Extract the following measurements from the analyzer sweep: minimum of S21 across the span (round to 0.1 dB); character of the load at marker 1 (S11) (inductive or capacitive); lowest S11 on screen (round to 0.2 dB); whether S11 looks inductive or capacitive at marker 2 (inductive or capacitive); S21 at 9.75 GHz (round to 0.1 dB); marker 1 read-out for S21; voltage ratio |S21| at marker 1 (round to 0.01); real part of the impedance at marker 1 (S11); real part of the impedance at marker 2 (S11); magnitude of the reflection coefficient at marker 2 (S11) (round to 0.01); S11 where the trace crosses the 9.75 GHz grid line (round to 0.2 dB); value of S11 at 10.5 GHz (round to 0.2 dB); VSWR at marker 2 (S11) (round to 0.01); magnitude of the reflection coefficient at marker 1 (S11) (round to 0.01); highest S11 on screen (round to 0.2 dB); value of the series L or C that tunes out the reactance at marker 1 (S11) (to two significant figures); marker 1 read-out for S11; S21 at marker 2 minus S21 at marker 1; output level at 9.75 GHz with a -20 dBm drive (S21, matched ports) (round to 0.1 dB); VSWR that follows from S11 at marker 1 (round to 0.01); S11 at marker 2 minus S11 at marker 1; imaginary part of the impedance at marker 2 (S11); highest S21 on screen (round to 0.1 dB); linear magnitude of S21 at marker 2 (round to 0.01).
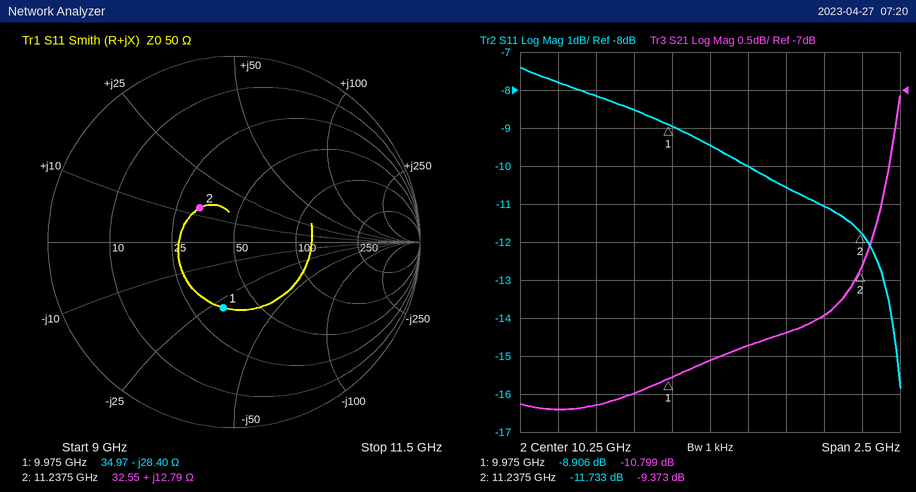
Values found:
-11.2 dB
capacitive
-15.8 dB
inductive
-11.0 dB
-10.799 dB
0.29
34.97 Ω
32.55 Ω
0.26
-8.6 dB
-10.0 dB
1.70
0.36
-7.4 dB
450 pH
-8.906 dB
1.426 dB
-31.0 dBm
2.12
-2.827 dB
+12.79 Ω
-7.1 dB
0.34
